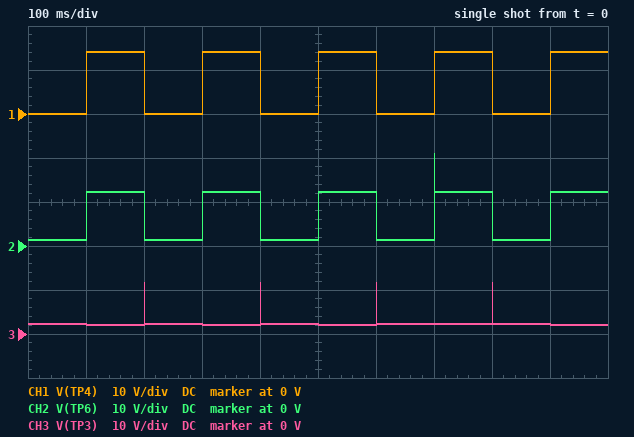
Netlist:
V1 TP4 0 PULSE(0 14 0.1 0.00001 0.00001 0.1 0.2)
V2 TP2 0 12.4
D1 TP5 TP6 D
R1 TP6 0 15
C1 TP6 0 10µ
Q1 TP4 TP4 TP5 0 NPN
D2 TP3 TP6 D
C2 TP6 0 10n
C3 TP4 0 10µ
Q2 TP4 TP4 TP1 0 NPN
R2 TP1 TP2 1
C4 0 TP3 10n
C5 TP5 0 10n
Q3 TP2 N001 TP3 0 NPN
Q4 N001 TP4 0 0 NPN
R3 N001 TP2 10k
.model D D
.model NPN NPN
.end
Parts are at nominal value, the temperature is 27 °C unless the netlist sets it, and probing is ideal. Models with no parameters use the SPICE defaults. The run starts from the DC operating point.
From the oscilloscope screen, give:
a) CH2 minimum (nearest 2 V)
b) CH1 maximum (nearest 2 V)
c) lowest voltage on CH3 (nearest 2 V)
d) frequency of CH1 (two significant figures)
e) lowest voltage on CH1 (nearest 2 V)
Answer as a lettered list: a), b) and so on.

a) 2 V
b) 14 V
c) 2 V
d) 5.0 Hz
e) 0 V
